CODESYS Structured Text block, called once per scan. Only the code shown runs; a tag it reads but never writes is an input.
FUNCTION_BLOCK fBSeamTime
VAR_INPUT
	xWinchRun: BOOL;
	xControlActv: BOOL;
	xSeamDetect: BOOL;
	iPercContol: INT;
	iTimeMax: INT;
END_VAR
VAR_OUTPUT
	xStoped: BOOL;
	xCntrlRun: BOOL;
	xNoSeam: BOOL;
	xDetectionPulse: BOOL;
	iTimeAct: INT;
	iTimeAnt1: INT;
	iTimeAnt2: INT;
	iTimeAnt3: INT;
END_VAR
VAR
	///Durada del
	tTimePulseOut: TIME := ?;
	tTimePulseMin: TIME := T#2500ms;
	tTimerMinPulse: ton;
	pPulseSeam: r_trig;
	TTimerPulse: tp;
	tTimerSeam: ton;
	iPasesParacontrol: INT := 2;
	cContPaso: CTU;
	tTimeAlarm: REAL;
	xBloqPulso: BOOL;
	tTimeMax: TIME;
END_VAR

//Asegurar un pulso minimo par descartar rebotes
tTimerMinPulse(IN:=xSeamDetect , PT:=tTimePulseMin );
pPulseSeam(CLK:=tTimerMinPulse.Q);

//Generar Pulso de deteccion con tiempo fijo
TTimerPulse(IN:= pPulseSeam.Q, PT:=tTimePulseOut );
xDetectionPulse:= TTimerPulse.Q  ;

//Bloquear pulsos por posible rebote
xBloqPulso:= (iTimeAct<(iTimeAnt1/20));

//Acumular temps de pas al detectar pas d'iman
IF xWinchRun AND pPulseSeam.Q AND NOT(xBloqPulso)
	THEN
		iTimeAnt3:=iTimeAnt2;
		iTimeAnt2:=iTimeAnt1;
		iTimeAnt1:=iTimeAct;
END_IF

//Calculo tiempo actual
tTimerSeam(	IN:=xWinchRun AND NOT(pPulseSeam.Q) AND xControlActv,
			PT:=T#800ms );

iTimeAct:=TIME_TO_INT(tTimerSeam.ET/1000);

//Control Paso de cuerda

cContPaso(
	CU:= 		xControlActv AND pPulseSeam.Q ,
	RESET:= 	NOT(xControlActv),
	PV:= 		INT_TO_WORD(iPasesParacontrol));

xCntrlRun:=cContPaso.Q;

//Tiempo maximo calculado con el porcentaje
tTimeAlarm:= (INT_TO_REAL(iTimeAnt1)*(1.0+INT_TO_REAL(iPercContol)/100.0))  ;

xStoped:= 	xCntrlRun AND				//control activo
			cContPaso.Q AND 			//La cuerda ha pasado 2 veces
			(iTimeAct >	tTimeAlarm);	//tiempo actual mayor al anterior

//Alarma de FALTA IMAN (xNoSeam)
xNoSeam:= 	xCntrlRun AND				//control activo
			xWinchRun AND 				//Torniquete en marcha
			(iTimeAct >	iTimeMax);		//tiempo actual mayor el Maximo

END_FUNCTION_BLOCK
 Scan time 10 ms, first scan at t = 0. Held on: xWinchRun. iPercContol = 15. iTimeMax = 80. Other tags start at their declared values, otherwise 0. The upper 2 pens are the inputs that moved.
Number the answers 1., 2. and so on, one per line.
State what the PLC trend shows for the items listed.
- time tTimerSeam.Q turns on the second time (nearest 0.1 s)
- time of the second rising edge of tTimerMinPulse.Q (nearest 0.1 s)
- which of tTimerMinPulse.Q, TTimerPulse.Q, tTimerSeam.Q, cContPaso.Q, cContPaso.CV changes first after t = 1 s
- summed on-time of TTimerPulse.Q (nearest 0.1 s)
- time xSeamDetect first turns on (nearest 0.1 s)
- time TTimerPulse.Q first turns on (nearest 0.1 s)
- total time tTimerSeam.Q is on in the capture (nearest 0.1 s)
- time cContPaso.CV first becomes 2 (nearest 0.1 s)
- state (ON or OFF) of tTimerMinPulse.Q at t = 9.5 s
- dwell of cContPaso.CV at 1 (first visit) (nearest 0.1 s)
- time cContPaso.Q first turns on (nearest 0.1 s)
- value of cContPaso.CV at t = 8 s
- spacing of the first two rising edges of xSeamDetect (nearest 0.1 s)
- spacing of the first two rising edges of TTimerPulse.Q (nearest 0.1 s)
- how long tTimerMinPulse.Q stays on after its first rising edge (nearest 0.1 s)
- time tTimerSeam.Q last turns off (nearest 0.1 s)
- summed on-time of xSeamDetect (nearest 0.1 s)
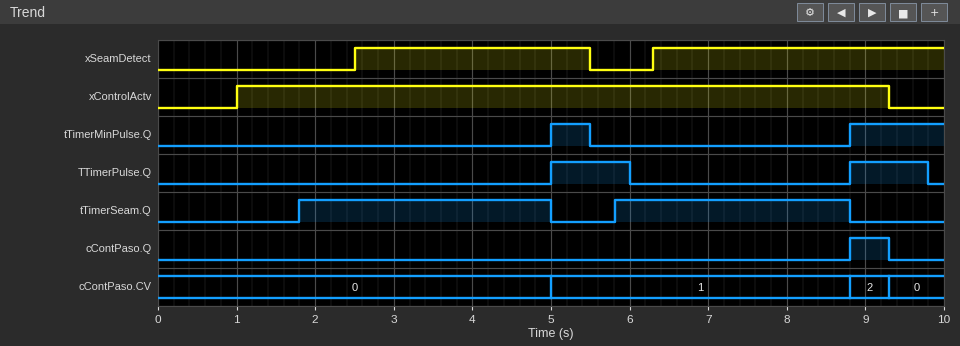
1. 5.8 s
2. 8.8 s
3. tTimerSeam.Q
4. 2.0 s
5. 2.5 s
6. 5.0 s
7. 6.2 s
8. 8.8 s
9. ON
10. 3.8 s
11. 8.8 s
12. 1
13. 3.8 s
14. 3.8 s
15. 0.5 s
16. 8.8 s
17. 6.7 s
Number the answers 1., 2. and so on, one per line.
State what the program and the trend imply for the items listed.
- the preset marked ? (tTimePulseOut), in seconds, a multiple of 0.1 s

1. 1.0 s
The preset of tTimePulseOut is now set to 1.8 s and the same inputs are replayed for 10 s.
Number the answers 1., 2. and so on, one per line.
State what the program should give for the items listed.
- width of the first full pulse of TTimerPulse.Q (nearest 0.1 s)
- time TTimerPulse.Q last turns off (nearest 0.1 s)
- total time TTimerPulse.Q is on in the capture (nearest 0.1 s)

1. 1.8 s
2. 6.8 s
3. 3.0 s
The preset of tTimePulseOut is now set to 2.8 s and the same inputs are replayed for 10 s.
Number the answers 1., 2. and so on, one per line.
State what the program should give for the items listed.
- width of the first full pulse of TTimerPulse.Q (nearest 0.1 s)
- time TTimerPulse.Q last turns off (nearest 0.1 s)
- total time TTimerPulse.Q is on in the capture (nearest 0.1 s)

1. 2.8 s
2. 7.8 s
3. 4.0 s
